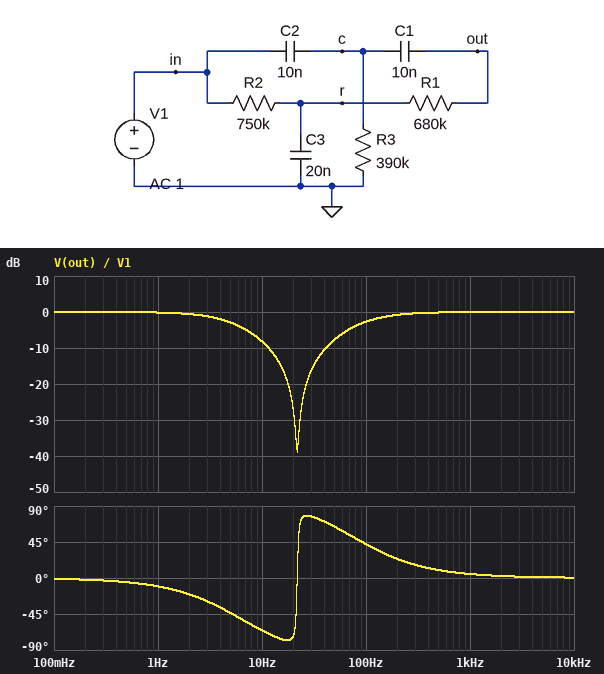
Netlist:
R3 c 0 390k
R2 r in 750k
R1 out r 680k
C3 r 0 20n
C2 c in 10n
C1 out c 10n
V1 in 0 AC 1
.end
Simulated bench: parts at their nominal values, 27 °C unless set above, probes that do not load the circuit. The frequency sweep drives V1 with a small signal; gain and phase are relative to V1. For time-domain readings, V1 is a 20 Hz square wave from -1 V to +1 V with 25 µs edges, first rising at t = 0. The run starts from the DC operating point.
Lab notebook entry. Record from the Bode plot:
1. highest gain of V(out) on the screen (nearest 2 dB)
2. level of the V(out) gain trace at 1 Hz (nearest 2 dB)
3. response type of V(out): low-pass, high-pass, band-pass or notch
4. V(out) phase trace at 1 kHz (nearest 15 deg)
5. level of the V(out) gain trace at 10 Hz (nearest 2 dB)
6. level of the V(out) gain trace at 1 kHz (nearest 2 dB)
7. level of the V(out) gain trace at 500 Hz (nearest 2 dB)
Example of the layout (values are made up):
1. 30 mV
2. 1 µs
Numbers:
1. 0 dB
2. 0 dB
3. notch
4. 0 deg
5. -8 dB
6. 0 dB
7. 0 dB
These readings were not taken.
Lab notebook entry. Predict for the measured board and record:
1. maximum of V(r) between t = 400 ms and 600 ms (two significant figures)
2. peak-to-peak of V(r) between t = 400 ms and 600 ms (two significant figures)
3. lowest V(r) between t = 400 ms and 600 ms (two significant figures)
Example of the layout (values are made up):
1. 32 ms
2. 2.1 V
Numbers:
1. 540 mV
2. 1.1 V
3. -540 mV
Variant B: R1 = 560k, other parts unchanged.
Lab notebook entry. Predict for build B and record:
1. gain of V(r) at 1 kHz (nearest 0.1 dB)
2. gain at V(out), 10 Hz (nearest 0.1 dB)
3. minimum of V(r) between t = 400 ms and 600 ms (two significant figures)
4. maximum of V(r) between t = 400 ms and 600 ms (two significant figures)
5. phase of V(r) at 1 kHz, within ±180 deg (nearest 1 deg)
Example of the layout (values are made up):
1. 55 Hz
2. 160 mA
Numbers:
1. -32.1 dB
2. -7.7 dB
3. -530 mV
4. 530 mV
5. -85 deg
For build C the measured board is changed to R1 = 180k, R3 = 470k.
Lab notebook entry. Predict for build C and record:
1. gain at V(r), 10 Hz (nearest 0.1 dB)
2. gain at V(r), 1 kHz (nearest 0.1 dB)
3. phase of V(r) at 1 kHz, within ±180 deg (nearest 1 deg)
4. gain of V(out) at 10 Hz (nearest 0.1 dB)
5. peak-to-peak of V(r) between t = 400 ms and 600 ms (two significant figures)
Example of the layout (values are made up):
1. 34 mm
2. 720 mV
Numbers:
1. -5.7 dB
2. -25.5 dB
3. -77 deg
4. -6.4 dB
5. 1.0 V
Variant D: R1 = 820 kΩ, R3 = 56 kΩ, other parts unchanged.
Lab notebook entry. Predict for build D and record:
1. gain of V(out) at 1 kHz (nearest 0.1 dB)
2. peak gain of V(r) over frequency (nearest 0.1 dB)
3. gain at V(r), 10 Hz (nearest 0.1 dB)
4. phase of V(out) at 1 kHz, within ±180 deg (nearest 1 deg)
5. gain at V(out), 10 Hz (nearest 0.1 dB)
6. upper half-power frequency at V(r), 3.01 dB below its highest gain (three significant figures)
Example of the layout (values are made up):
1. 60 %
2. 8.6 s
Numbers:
1. -0.4 dB
2. 0 dB
3. -5.1 dB
4. 18 deg
5. -6.4 dB
6. 6.47 Hz
